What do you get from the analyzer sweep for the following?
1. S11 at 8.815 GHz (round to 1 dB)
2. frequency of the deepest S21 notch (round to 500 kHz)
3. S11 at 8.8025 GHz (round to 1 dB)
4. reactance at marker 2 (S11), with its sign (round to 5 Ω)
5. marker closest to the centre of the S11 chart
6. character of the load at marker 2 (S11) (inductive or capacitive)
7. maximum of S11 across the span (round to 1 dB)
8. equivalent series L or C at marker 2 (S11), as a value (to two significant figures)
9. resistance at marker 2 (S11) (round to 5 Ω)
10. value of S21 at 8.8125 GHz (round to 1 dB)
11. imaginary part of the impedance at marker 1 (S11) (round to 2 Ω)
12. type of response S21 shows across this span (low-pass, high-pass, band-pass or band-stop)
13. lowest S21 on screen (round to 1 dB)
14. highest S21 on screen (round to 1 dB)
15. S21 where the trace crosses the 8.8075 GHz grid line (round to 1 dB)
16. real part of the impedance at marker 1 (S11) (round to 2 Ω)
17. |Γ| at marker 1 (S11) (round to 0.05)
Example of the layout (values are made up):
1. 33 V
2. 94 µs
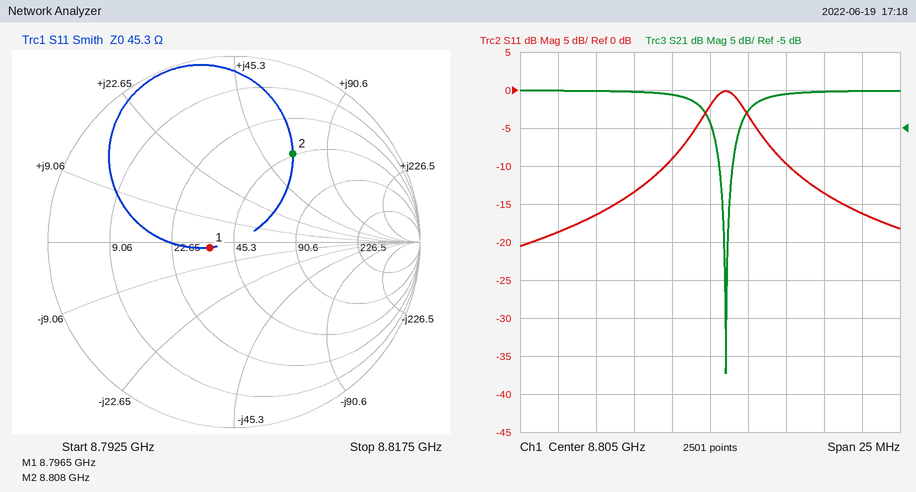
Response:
1. -16 dB
2. 8.8060 GHz
3. -9 dB
4. +60 Ω
5. marker 1
6. inductive
7. 0 dB
8. 1.1 nH
9. 45 Ω
10. 0 dB
11. -2 Ω
12. band-stop
13. -37 dB
14. 0 dB
15. -3 dB
16. 34 Ω
17. 0.15
